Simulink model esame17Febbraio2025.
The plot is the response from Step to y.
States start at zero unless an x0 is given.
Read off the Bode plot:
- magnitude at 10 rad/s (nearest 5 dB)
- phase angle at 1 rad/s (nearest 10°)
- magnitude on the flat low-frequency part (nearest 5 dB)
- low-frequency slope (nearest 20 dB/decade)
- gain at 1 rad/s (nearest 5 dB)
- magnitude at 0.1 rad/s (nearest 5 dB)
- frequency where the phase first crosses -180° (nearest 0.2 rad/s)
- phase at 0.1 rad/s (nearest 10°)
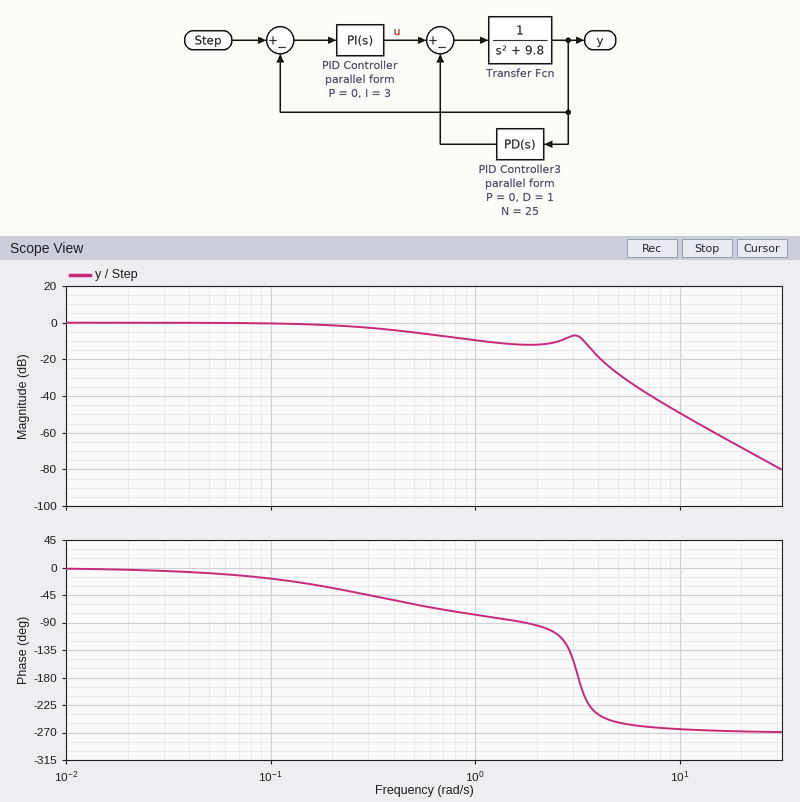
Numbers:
-50 dB
-80°
0 dB
0 dB/decade
-10 dB
0 dB
3.2 rad/s
-20°
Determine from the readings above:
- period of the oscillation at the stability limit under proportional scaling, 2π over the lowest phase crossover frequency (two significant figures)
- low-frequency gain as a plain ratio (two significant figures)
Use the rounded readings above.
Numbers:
2.0 s
1.0
